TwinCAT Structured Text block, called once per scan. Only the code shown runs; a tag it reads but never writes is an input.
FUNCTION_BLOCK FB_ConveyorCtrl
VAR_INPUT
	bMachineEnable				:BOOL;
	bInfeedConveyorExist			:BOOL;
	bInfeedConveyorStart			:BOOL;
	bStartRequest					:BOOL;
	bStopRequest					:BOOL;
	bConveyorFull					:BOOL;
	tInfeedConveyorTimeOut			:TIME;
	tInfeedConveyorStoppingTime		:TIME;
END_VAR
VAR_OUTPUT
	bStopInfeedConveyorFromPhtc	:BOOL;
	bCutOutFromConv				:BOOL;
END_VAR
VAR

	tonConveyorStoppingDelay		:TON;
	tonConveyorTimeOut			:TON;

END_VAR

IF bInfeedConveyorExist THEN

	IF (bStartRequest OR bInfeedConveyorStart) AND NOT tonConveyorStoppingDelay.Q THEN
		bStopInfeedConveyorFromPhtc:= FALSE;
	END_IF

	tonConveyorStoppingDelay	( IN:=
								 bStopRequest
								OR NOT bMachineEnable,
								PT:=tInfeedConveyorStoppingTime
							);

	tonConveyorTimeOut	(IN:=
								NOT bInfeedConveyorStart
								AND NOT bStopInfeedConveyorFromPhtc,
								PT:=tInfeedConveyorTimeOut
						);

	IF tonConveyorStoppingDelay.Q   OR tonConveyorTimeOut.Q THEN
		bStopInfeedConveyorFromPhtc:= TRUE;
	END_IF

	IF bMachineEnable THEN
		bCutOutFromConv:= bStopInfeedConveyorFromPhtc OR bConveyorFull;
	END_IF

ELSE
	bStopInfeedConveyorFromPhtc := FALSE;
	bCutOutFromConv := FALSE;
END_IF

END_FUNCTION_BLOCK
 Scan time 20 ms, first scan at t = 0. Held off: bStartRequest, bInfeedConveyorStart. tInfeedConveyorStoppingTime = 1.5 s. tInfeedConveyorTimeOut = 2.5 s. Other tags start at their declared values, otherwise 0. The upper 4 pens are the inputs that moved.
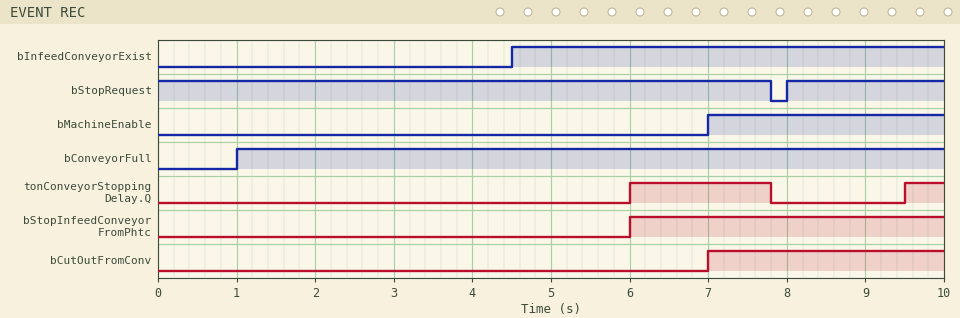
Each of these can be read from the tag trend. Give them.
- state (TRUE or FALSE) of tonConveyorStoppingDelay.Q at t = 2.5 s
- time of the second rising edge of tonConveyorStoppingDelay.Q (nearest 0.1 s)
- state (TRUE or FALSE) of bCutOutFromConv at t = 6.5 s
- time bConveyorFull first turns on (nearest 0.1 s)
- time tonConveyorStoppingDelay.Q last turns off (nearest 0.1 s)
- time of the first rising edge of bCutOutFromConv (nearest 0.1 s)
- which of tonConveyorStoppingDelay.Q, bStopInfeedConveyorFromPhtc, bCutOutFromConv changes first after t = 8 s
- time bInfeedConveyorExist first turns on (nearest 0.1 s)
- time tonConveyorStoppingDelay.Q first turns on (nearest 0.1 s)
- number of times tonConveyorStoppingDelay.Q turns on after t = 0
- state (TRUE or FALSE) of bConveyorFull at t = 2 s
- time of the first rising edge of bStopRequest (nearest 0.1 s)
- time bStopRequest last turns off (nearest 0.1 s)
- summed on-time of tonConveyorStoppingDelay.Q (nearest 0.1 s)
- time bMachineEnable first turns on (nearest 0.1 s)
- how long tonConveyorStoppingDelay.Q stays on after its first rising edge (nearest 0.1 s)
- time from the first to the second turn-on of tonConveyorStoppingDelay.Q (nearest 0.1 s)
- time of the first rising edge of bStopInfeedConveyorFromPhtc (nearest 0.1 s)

FALSE
9.5 s
FALSE
1.0 s
7.8 s
7.0 s
tonConveyorStoppingDelay.Q
4.5 s
6.0 s
2
TRUE
8.0 s
7.8 s
2.3 s
7.0 s
1.8 s
3.5 s
6.0 s
